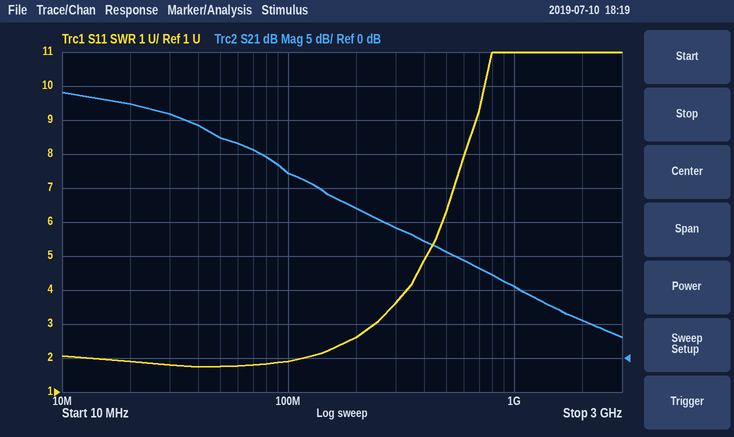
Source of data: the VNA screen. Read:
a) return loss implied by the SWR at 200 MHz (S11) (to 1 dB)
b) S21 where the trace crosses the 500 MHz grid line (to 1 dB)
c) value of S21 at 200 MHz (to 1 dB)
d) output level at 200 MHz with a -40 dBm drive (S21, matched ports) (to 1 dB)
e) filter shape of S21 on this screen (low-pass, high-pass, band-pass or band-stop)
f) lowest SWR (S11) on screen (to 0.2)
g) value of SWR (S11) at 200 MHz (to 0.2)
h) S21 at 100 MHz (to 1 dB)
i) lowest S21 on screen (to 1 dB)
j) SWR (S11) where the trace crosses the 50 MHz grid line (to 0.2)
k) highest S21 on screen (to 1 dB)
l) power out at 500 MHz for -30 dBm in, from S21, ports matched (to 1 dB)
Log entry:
7 dB
16 dB
22 dB
-18 dBm
low-pass
1.8
2.6
27 dB
3 dB
1.8
39 dB
-14 dBm
